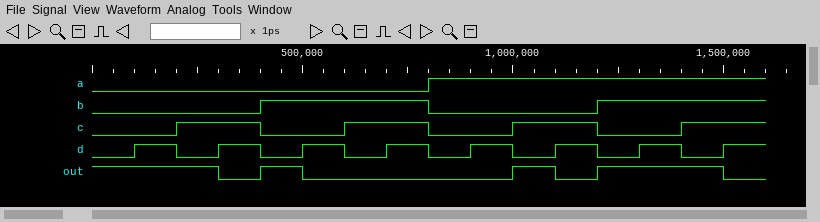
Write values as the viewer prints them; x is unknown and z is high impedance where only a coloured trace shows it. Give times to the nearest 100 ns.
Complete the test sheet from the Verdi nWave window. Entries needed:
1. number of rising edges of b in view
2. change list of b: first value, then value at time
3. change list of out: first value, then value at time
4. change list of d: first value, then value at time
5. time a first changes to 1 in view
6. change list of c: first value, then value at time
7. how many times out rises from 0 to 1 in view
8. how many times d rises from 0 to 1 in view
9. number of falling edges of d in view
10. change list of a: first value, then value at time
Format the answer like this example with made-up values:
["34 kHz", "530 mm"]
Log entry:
["2", "0, 1 at 400 ns, 0 at 800 ns, 1 at 1200 ns", "1, 0 at 300 ns, 1 at 400 ns, 0 at 500 ns, 1 at 1000 ns, 0 at 1100 ns, 1 at 1200 ns, 0 at 1500 ns", "0, 1 at 100 ns, 0 at 200 ns, 1 at 300 ns, 0 at 400 ns, 1 at 500 ns, 0 at 600 ns, 1 at 700 ns, 0 at 800 ns, 1 at 900 ns, 0 at 1000 ns, 1 at 1100 ns, 0 at 1200 ns, 1 at 1300 ns, 0 at 1400 ns, 1 at 1500 ns", "800 ns", "0, 1 at 200 ns, 0 at 400 ns, 1 at 600 ns, 0 at 800 ns, 1 at 1000 ns, 0 at 1200 ns, 1 at 1400 ns", "3", "8", "7", "0, 1 at 800 ns"]
